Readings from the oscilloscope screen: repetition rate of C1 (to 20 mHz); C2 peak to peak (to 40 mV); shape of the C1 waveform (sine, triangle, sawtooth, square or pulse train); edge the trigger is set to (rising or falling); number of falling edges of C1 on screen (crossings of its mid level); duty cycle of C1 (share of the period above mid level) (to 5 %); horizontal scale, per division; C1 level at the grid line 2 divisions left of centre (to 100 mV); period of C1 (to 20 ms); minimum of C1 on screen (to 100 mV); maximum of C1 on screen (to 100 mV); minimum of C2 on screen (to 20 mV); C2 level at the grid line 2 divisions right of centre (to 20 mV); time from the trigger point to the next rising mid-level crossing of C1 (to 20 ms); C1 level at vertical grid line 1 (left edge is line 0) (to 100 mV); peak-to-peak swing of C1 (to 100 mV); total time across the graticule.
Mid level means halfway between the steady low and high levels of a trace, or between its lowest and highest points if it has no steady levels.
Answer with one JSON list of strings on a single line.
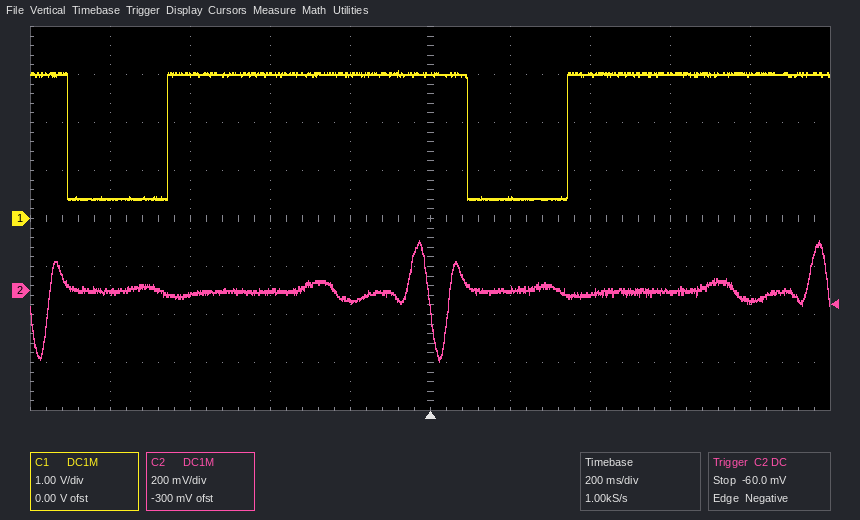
["1.00 Hz", "520 mV", "pulse train", "falling", "2", "75 %", "200 ms", "3.0 V", "1.00 s", "400 mV", "3.1 V", "-300 mV", "-20 mV", "340 ms", "400 mV", "2.7 V", "2 s"]
